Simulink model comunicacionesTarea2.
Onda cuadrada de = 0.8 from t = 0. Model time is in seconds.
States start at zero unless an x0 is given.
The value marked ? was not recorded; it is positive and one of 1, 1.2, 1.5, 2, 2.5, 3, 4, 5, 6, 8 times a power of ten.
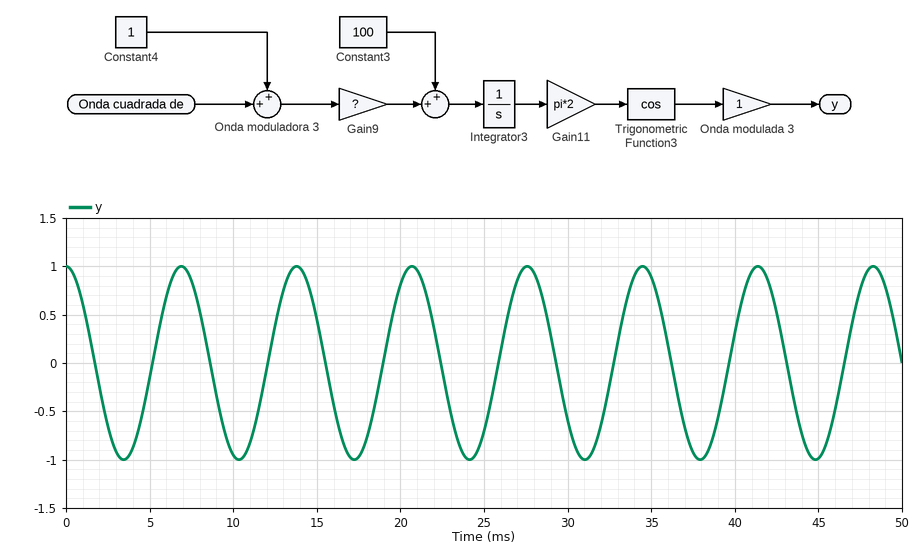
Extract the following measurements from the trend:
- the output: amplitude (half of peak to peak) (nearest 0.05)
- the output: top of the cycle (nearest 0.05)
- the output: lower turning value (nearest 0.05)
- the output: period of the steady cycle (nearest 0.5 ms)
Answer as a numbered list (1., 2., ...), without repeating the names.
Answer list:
1. 1.00
2. 1.00
3. -1.00
4. 7.0 ms
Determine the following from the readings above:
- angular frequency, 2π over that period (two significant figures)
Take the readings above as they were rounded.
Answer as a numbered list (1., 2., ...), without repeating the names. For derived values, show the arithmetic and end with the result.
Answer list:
1. 2π / 7 = 0.90 rad/ms
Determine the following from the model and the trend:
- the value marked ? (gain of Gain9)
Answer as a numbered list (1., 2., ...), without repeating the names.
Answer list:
1. 25
